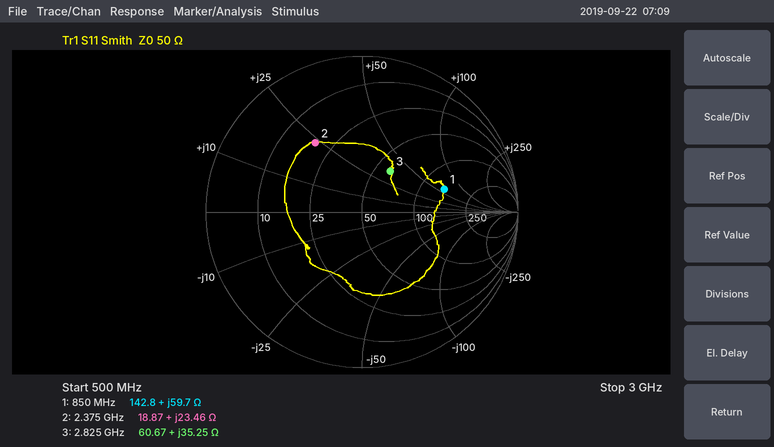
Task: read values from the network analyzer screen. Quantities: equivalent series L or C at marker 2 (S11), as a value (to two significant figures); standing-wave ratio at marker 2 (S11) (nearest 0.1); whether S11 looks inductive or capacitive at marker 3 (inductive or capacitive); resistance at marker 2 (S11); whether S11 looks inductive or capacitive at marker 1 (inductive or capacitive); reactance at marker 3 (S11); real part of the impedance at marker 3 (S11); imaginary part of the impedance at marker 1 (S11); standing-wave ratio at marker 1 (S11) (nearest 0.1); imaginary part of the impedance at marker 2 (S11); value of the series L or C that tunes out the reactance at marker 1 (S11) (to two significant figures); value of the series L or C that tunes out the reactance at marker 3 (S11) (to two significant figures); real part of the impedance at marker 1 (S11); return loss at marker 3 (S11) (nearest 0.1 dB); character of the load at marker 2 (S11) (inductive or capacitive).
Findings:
1.6 nH
3.3
inductive
18.87 Ω
inductive
+35.25 Ω
60.67 Ω
+59.7 Ω
3.4
+23.46 Ω
3.1 pF
1.6 pF
142.8 Ω
10.0 dB
inductive
